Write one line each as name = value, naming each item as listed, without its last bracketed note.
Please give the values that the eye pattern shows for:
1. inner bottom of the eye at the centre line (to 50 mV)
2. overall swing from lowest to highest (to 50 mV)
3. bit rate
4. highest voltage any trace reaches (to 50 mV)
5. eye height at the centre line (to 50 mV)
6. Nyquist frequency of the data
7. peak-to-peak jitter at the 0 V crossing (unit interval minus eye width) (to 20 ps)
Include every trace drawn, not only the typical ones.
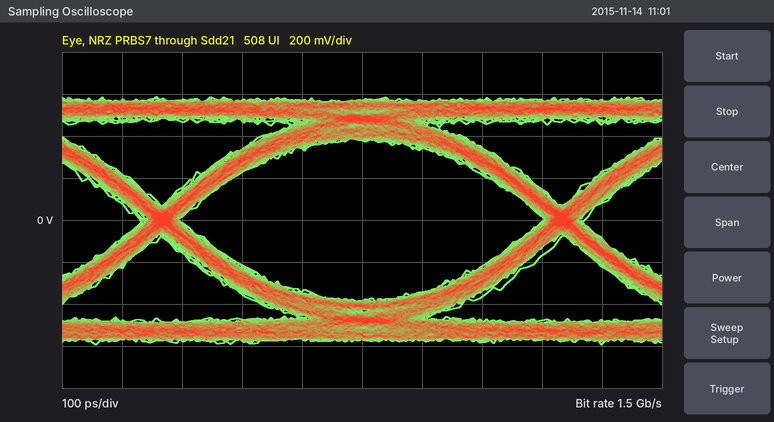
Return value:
inner bottom of the eye at the centre line = -400 mV
overall swing from lowest to highest = 1.20 V
bit rate = 1.5 Gb/s
highest voltage any trace reaches = 600 mV
eye height at the centre line = 750 mV
Nyquist frequency of the data = 750 MHz
peak-to-peak jitter at the 0 V crossing (unit interval minus eye width) = 60 ps
